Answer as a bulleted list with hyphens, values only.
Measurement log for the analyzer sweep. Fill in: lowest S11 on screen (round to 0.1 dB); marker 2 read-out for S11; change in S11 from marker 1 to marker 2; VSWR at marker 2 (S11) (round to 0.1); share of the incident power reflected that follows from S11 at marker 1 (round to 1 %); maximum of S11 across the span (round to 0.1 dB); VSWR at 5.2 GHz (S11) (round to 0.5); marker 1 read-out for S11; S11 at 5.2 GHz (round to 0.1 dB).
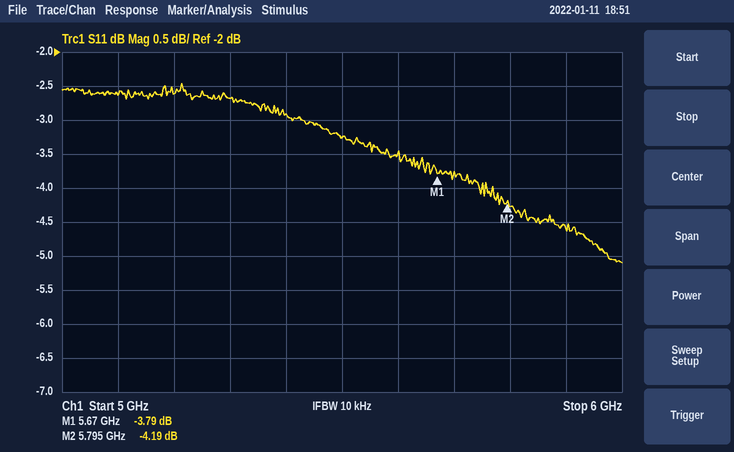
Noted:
- -5.1 dB
- -4.19 dB
- -0.40 dB
- 4.2
- 42 %
- -2.5 dB
- 6.5
- -3.79 dB
- -2.6 dB
